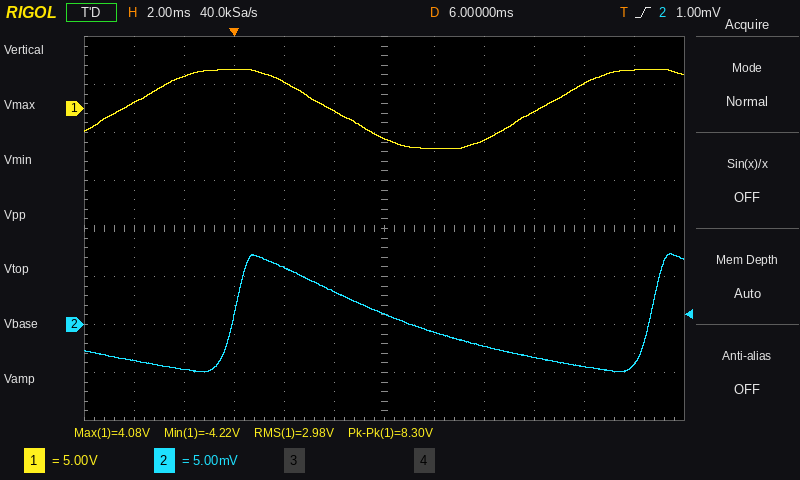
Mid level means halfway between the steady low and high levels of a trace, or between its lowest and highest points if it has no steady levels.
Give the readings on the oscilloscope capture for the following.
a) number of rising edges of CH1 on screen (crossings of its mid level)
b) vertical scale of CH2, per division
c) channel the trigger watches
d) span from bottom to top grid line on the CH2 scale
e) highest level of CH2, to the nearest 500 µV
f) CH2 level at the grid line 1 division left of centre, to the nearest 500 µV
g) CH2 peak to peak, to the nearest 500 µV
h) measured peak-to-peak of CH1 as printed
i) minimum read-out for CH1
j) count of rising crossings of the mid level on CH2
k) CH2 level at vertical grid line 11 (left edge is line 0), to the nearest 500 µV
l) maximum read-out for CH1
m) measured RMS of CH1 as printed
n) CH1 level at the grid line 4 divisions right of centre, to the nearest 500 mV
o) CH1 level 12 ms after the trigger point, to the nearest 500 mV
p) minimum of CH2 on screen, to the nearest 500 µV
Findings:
2
5 mV
CH2
40 mV
7.5 mV
3.5 mV
12.5 mV
8.30 V
-4.22 V
2
-4.0 mV
4.08 V
2.98 V
2.5 V
-500 mV
-5.0 mV
